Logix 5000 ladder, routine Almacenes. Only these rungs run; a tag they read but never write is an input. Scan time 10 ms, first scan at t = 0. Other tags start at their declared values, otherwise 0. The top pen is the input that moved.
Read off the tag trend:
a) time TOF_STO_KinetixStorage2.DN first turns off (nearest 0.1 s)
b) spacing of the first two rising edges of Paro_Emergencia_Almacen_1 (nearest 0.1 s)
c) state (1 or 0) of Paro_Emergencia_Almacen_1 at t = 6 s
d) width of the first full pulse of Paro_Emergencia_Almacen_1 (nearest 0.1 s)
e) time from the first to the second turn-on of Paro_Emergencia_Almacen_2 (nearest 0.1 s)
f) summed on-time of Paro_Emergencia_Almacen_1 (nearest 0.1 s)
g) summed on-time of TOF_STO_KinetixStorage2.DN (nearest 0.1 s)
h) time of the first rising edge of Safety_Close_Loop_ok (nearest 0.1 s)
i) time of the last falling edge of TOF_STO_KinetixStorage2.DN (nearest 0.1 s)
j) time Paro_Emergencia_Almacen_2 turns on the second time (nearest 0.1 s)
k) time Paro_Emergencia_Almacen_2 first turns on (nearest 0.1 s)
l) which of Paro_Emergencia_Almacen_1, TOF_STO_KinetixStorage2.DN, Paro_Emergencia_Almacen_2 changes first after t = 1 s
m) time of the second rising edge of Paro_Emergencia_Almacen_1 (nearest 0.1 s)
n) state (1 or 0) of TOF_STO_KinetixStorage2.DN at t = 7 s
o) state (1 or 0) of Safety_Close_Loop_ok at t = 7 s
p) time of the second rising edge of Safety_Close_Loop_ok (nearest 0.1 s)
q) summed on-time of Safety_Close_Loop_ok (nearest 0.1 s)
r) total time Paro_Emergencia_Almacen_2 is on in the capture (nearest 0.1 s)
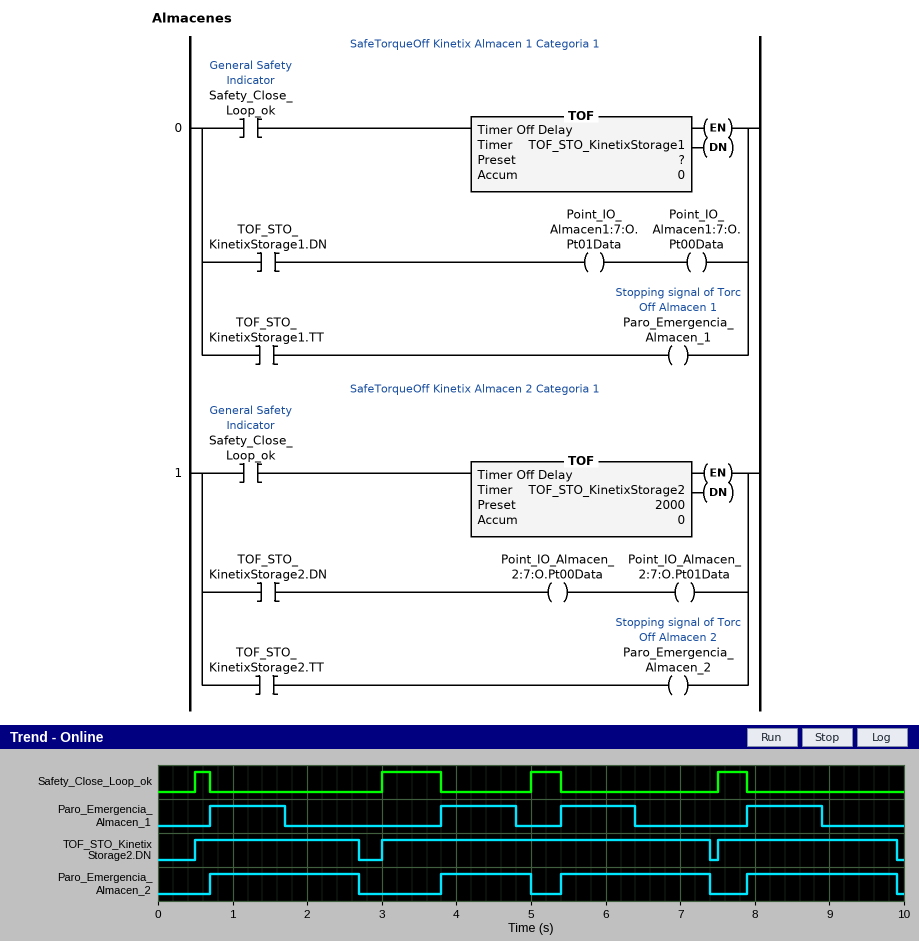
2.7 s
3.1 s
1
1.0 s
3.1 s
4.0 s
9.0 s
0.5 s
9.9 s
3.8 s
0.7 s
Paro_Emergencia_Almacen_1
3.8 s
1
0
3.0 s
1.8 s
7.2 s
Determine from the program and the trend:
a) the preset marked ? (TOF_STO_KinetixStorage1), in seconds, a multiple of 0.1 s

1.0 s
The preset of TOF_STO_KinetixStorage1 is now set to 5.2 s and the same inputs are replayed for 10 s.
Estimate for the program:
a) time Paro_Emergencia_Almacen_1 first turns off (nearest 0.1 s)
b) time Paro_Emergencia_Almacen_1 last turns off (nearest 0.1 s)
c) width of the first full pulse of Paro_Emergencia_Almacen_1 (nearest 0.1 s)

3.0 s
7.5 s
2.3 s
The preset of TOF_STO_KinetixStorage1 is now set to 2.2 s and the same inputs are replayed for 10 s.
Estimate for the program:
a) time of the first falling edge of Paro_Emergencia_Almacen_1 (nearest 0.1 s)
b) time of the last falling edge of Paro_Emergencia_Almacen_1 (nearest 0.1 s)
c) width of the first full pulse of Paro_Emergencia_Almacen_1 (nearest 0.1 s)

2.9 s
7.5 s
2.2 s
